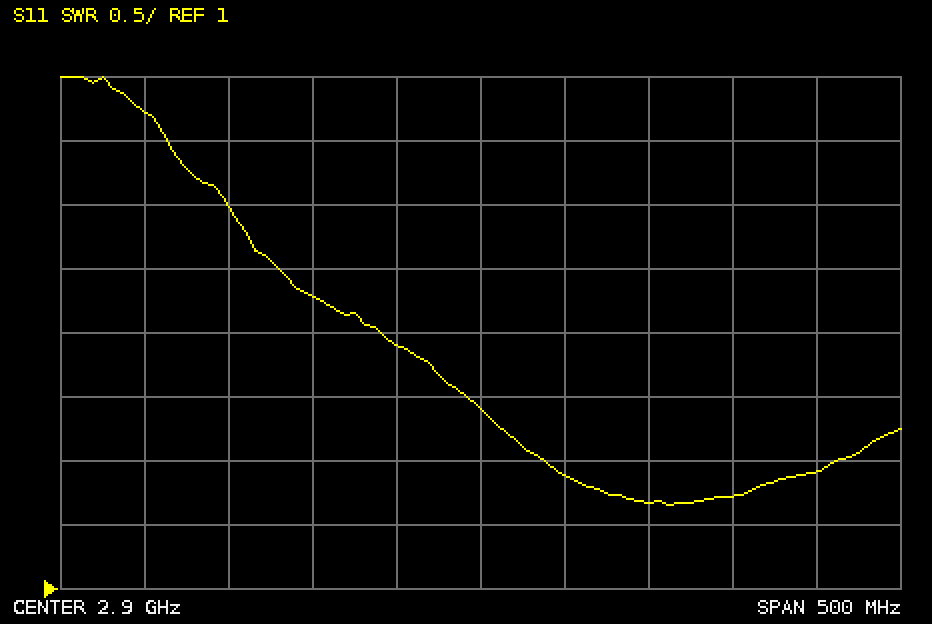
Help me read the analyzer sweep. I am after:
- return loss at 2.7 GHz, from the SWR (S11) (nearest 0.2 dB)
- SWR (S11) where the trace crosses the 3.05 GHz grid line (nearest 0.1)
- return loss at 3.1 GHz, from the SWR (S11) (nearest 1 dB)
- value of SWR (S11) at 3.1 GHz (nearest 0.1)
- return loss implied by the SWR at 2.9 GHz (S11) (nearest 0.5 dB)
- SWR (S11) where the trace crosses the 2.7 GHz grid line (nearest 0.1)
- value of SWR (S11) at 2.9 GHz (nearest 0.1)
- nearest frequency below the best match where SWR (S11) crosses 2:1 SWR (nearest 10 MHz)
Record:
3.8 dB
1.7
10 dB
1.9
7.5 dB
4.7
2.4
2.94 GHz
